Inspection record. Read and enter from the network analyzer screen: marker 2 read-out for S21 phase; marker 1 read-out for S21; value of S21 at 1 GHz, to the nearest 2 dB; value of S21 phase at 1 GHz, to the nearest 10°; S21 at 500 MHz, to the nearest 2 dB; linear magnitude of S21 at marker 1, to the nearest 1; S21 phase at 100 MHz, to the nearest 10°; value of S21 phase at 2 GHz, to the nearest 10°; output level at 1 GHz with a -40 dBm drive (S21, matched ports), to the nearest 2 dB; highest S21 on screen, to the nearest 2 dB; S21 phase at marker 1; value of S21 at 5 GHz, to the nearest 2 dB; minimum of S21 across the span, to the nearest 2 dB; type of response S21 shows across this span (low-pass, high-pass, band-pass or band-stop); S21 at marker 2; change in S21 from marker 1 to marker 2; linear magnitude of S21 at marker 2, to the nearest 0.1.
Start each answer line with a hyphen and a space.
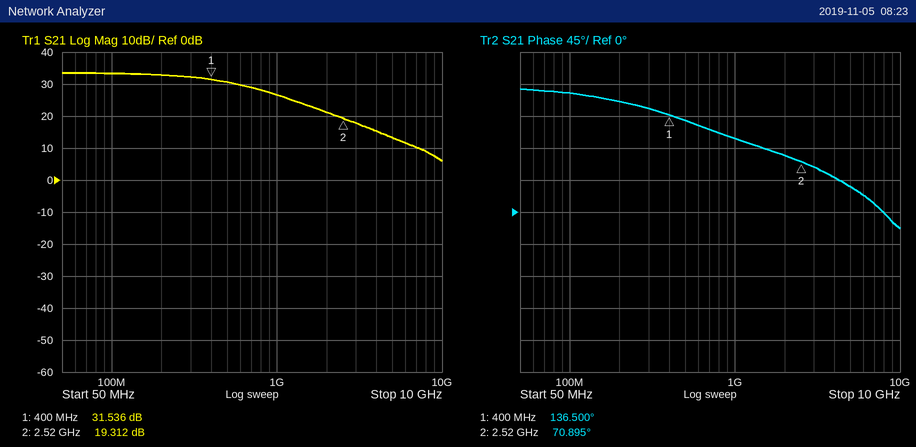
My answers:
- 70.895°
- 31.536 dB
- 26 dB
- 100°
- 30 dB
- 38
- 170°
- 80°
- -14 dBm
- 34 dB
- 136.500°
- 14 dB
- 6 dB
- low-pass
- 19.312 dB
- -12.224 dB
- 9.2
